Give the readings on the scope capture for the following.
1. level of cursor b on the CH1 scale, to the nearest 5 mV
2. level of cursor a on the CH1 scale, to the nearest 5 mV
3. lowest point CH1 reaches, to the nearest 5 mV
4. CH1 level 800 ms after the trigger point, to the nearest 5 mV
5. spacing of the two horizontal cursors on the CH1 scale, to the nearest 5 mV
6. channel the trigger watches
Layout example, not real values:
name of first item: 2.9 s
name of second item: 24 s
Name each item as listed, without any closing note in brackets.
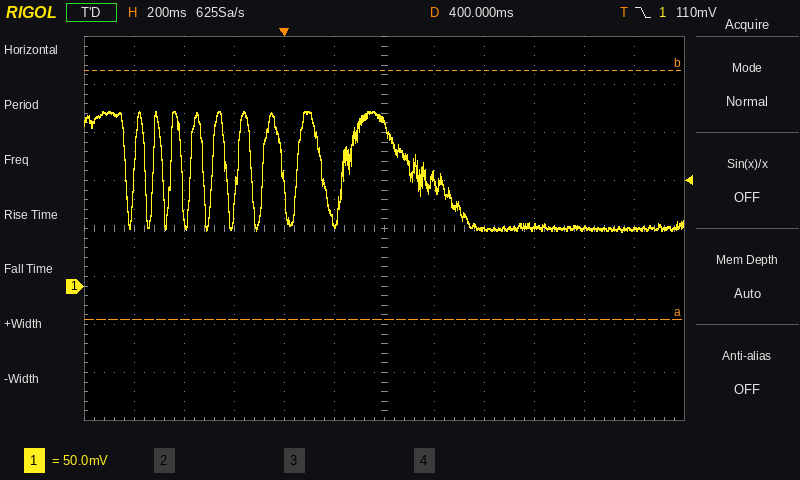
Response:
level of cursor b on the CH1 scale, to the nearest 5 mV: 225 mV
level of cursor a on the CH1 scale, to the nearest 5 mV: -35 mV
lowest point CH1 reaches, to the nearest 5 mV: 55 mV
CH1 level 800 ms after the trigger point, to the nearest 5 mV: 60 mV
spacing of the two horizontal cursors on the CH1 scale, to the nearest 5 mV: 260 mV
channel the trigger watches: CH1
